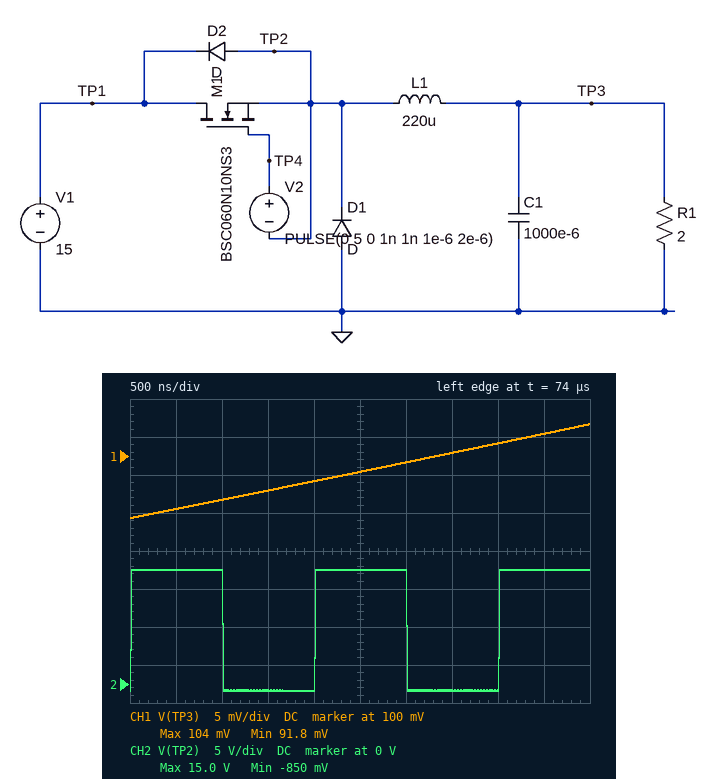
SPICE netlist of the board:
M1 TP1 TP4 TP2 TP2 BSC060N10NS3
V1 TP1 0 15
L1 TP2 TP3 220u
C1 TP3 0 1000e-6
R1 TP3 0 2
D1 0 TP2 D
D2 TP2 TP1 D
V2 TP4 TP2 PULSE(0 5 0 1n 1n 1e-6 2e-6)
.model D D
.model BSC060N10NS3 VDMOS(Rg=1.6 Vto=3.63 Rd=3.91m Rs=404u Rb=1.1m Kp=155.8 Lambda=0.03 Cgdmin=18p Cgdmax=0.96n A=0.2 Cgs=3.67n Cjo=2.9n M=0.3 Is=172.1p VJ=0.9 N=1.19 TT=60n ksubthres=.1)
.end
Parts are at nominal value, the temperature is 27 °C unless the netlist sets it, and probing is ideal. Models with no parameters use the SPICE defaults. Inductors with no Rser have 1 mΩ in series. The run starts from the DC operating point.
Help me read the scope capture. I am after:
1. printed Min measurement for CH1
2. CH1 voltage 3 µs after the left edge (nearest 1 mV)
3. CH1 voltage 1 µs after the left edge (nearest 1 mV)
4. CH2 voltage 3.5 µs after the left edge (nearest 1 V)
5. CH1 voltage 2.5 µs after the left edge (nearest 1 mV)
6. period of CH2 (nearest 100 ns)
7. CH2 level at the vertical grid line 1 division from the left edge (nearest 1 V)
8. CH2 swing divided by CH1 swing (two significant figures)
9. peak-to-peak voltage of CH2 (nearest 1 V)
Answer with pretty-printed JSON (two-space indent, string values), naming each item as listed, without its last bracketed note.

{
  "printed Min measurement for CH1": "91.8 mV",
  "CH1 voltage 3 µs after the left edge": "99 mV",
  "CH1 voltage 1 µs after the left edge": "94 mV",
  "CH2 voltage 3.5 µs after the left edge": "-1 V",
  "CH1 voltage 2.5 µs after the left edge": "98 mV",
  "period of CH2": "2.0 µs",
  "CH2 level at the vertical grid line 1 division from the left edge": "15 V",
  "CH2 swing divided by CH1 swing": "1300",
  "peak-to-peak voltage of CH2": "16 V"
}
